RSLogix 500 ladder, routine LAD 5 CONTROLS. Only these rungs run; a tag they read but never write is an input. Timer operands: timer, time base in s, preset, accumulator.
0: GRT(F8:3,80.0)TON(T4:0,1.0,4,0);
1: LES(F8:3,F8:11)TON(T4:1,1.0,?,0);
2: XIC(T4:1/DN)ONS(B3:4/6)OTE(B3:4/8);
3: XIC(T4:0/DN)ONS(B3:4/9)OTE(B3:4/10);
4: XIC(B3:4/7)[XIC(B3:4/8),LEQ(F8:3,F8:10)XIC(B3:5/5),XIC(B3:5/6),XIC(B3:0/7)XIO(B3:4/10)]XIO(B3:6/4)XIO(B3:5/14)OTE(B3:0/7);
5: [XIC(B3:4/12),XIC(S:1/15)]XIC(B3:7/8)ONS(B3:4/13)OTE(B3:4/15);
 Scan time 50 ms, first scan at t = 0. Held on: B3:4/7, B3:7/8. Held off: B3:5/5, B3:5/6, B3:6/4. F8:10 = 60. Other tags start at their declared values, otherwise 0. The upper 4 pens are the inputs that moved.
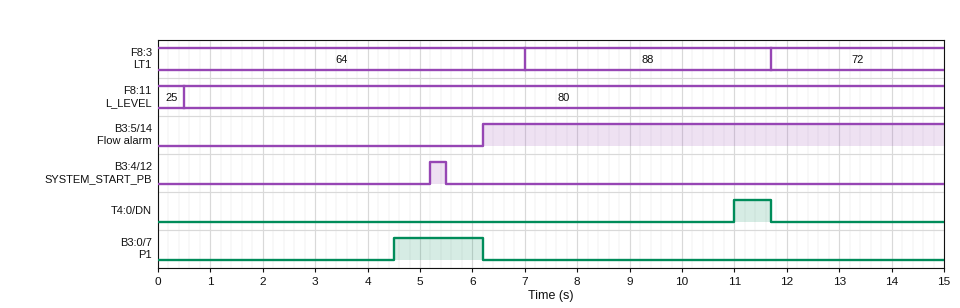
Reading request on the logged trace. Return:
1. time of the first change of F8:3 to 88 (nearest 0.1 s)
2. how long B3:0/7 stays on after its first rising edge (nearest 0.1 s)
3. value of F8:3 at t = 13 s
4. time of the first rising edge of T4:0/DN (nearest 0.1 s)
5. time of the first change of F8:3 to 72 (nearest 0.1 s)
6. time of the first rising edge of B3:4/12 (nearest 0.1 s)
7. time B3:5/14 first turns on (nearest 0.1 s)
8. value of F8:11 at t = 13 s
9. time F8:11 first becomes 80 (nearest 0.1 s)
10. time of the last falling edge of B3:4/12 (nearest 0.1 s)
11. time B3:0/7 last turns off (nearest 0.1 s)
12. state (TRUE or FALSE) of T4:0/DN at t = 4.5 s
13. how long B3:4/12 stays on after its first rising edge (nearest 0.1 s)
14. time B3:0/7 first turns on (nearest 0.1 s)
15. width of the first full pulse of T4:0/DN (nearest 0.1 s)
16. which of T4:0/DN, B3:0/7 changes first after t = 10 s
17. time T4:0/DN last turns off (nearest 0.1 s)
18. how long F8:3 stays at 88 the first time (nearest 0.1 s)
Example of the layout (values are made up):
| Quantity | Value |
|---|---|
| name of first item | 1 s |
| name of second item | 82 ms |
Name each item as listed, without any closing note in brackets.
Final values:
| Quantity | Value |
|---|---|
| time of the first change of F8:3 to 88 | 7.0 s |
| how long B3:0/7 stays on after its first rising edge | 1.7 s |
| value of F8:3 at t = 13 s | 72 |
| time of the first rising edge of T4:0/DN | 11.0 s |
| time of the first change of F8:3 to 72 | 11.7 s |
| time of the first rising edge of B3:4/12 | 5.2 s |
| time B3:5/14 first turns on | 6.2 s |
| value of F8:11 at t = 13 s | 80 |
| time F8:11 first becomes 80 | 0.5 s |
| time of the last falling edge of B3:4/12 | 5.5 s |
| time B3:0/7 last turns off | 6.2 s |
| state (TRUE or FALSE) of T4:0/DN at t = 4.5 s | FALSE |
| how long B3:4/12 stays on after its first rising edge | 0.3 s |
| time B3:0/7 first turns on | 4.5 s |
| width of the first full pulse of T4:0/DN | 0.7 s |
| which of T4:0/DN, B3:0/7 changes first after t = 10 s | T4:0/DN |
| time T4:0/DN last turns off | 11.7 s |
| how long F8:3 stays at 88 the first time | 4.7 s |
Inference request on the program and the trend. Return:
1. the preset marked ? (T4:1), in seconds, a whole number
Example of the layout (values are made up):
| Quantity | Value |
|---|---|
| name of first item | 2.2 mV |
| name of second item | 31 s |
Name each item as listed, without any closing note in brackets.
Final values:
| Quantity | Value |
|---|---|
| the preset marked ? (T4:1), in seconds, a whole number | 4 s |
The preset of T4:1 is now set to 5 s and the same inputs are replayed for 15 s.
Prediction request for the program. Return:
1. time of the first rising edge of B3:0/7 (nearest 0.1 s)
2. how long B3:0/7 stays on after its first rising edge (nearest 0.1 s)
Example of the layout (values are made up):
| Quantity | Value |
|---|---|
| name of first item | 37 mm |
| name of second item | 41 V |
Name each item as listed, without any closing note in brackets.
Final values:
| Quantity | Value |
|---|---|
| time of the first rising edge of B3:0/7 | 5.5 s |
| how long B3:0/7 stays on after its first rising edge | 0.7 s |
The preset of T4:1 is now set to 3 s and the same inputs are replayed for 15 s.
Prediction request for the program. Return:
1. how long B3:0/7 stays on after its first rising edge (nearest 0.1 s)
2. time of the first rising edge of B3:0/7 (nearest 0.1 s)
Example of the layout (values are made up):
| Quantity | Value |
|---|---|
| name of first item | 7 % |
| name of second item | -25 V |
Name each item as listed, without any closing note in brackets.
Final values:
| Quantity | Value |
|---|---|
| how long B3:0/7 stays on after its first rising edge | 2.7 s |
| time of the first rising edge of B3:0/7 | 3.5 s |
